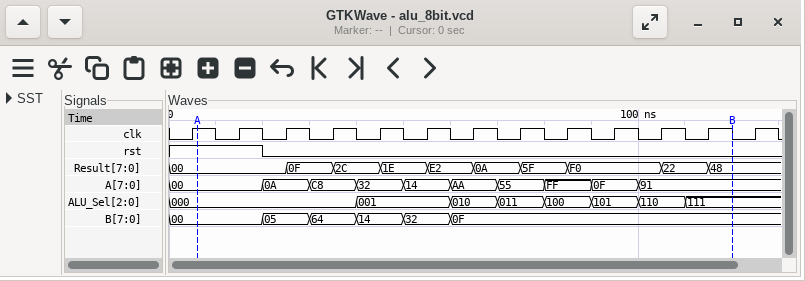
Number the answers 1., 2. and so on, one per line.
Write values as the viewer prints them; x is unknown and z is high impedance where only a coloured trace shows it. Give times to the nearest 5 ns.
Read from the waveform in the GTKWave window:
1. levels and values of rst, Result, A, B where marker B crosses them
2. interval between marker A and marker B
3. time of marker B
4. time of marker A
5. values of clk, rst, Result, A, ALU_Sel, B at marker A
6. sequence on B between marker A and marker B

1. rst=0, Result=48, A=91, B=0F
2. 115 ns
3. 120 ns
4. 5 ns
5. clk=1, rst=1, Result=00, A=00, ALU_Sel=000, B=00
6. 00, 05, 64, 14, 32, 0F
